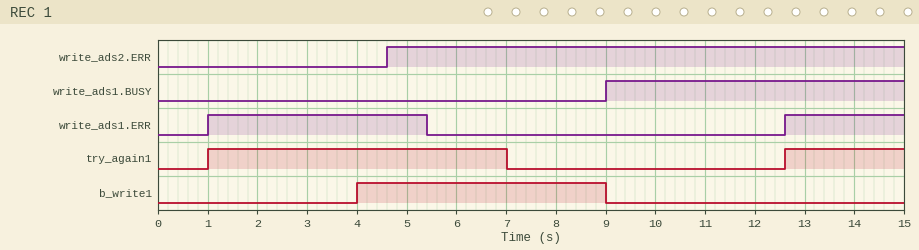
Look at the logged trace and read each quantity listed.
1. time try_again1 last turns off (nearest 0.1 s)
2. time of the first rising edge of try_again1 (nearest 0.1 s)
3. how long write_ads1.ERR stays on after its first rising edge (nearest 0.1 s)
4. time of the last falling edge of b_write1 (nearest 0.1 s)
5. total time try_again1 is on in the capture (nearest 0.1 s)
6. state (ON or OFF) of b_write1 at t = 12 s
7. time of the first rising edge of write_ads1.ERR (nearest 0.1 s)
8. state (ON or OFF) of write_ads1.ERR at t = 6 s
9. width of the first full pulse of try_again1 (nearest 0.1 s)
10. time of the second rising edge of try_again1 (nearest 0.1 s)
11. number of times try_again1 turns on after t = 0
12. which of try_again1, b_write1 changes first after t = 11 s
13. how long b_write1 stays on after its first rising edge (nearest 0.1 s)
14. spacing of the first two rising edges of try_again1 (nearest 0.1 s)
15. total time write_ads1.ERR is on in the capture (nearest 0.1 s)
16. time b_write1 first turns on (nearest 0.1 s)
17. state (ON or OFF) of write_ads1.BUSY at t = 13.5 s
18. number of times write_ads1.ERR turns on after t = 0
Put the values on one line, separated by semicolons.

7.0 s; 1.0 s; 4.4 s; 9.0 s; 8.4 s; OFF; 1.0 s; OFF; 6.0 s; 12.6 s; 2; try_again1; 5.0 s; 11.6 s; 6.8 s; 4.0 s; ON; 2
